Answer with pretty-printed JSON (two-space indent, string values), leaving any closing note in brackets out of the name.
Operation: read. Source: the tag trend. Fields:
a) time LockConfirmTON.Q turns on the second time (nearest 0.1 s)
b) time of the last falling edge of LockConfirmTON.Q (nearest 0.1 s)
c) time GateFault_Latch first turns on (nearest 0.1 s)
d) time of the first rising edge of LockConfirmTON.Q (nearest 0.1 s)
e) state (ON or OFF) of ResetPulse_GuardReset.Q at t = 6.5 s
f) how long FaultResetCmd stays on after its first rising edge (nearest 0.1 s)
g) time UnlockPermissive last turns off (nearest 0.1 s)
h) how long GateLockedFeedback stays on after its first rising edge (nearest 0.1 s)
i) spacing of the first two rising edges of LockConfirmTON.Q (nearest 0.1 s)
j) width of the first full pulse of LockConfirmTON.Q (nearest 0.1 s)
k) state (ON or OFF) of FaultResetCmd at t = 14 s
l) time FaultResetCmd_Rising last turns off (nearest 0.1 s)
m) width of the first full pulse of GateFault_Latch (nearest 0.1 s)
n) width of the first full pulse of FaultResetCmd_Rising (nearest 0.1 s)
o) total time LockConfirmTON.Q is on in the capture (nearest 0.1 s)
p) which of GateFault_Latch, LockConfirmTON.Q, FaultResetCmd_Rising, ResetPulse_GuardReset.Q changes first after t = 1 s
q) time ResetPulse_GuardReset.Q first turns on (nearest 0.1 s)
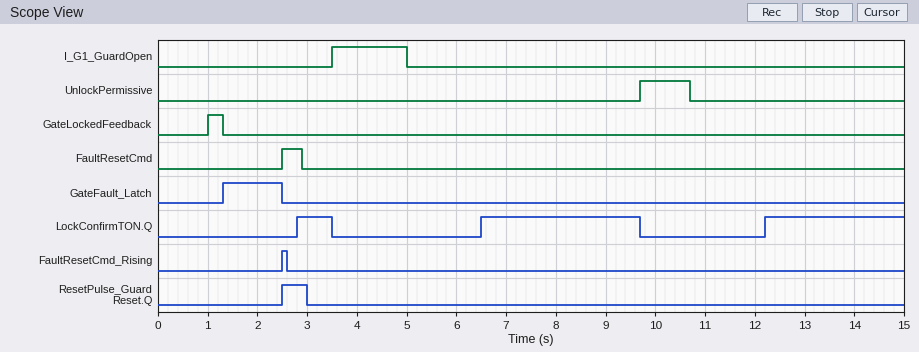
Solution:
{
  "time LockConfirmTON.Q turns on the second time": "6.5 s",
  "time of the last falling edge of LockConfirmTON.Q": "9.7 s",
  "time GateFault_Latch first turns on": "1.3 s",
  "time of the first rising edge of LockConfirmTON.Q": "2.8 s",
  "state (ON or OFF) of ResetPulse_GuardReset.Q at t = 6.5 s": "OFF",
  "how long FaultResetCmd stays on after its first rising edge": "0.4 s",
  "time UnlockPermissive last turns off": "10.7 s",
  "how long GateLockedFeedback stays on after its first rising edge": "0.3 s",
  "spacing of the first two rising edges of LockConfirmTON.Q": "3.7 s",
  "width of the first full pulse of LockConfirmTON.Q": "0.7 s",
  "state (ON or OFF) of FaultResetCmd at t = 14 s": "OFF",
  "time FaultResetCmd_Rising last turns off": "2.6 s",
  "width of the first full pulse of GateFault_Latch": "1.2 s",
  "width of the first full pulse of FaultResetCmd_Rising": "0.1 s",
  "total time LockConfirmTON.Q is on in the capture": "6.7 s",
  "which of GateFault_Latch, LockConfirmTON.Q, FaultResetCmd_Rising, ResetPulse_GuardReset.Q changes first after t = 1 s": "GateFault_Latch",
  "time ResetPulse_GuardReset.Q first turns on": "2.5 s"
}
